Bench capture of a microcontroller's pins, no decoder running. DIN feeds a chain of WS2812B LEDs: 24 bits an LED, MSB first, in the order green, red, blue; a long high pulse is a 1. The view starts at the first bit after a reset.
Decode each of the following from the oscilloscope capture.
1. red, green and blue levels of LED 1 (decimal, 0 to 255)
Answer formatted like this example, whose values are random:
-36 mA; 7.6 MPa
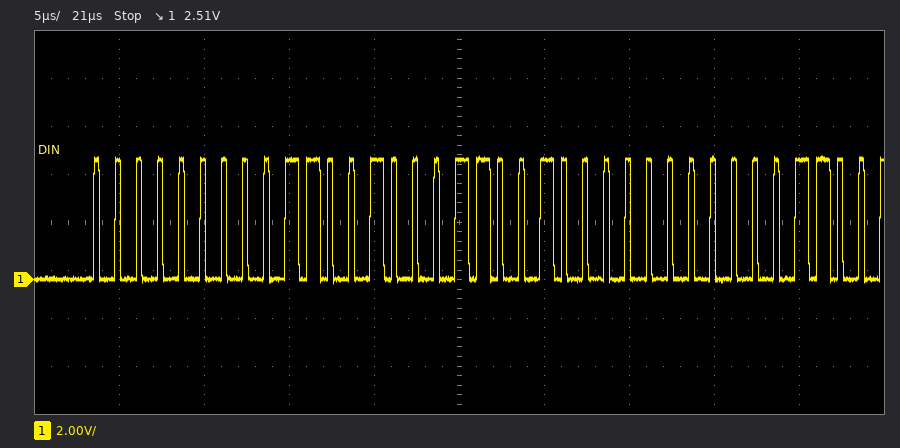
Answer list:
100, 0, 100
